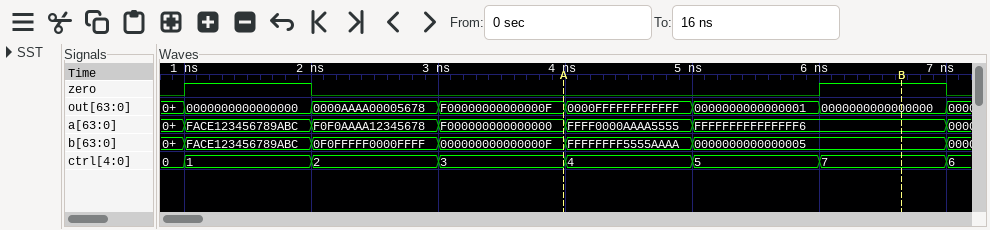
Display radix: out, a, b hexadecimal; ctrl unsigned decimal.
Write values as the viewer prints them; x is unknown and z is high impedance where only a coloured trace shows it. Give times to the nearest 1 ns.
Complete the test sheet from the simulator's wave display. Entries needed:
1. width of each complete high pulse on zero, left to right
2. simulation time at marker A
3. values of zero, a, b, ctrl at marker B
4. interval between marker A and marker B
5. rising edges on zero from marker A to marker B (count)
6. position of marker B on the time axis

1 ns, 1 ns
4 ns
zero=1, a=FFFFFFFFFFFFFFF6, b=0000000000000005, ctrl=7
3 ns
1
7 ns
